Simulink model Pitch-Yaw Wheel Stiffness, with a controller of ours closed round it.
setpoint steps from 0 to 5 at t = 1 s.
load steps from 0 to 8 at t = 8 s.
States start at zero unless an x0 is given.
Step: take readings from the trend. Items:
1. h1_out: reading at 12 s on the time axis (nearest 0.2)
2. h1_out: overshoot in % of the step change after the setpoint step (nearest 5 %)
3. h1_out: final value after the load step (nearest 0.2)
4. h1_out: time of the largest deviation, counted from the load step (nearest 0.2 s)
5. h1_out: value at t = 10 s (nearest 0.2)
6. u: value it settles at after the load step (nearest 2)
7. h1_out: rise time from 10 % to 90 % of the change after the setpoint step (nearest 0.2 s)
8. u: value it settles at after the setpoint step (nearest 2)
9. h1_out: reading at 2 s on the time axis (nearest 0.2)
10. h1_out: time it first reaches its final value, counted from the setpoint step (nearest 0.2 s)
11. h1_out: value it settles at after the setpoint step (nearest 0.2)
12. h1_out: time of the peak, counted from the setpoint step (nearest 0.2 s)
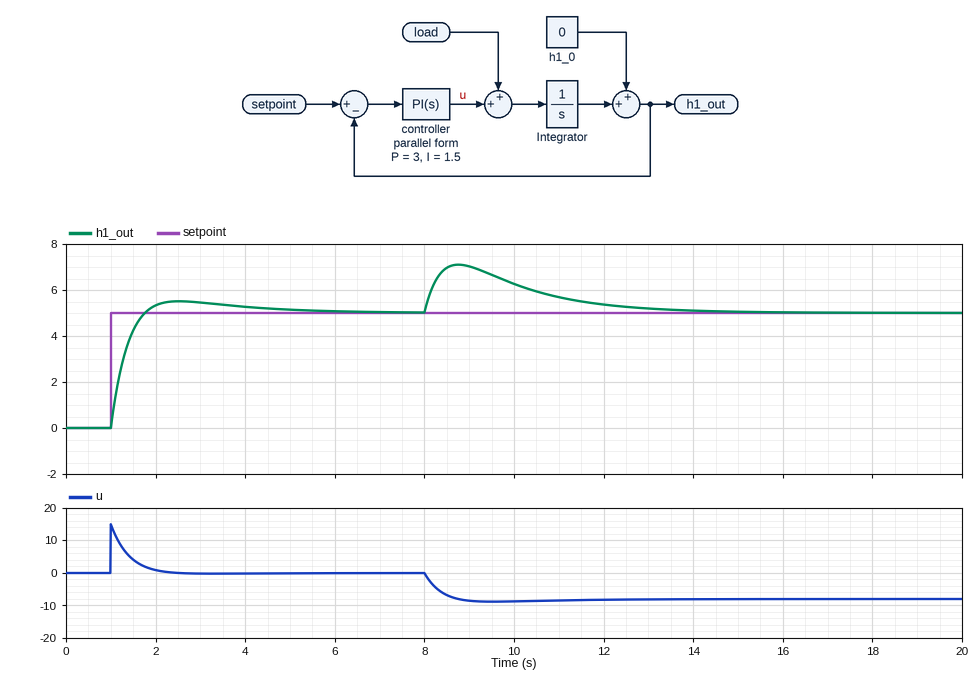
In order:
5.4
10 %
5.0
0.8 s
6.2
-8
0.6 s
0
5.4
0.8 s
5.0
1.6 s
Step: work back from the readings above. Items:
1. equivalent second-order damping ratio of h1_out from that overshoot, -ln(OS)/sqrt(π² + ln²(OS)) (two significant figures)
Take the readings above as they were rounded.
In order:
0.59
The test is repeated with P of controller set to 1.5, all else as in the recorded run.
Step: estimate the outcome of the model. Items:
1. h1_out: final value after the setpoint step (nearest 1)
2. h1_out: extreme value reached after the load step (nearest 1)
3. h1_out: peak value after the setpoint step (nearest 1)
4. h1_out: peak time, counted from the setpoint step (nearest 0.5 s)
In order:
5
8
6
2.0 s
